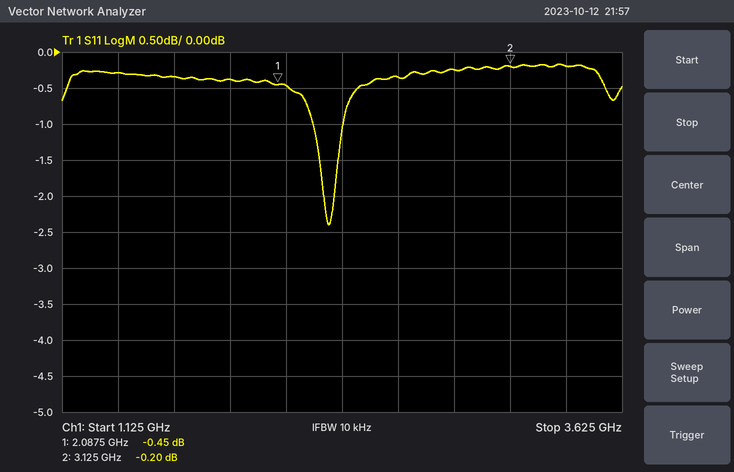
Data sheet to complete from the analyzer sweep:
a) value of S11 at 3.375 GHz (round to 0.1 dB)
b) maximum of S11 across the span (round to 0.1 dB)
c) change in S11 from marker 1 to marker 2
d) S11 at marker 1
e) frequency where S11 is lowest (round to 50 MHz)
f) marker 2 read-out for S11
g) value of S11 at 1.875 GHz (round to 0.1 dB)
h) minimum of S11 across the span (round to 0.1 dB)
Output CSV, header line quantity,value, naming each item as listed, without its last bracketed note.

quantity,value
value of S11 at 3.375 GHz,-0.2 dB
maximum of S11 across the span,-0.2 dB
change in S11 from marker 1 to marker 2,0.25 dB
S11 at marker 1,-0.45 dB
frequency where S11 is lowest,2.30 GHz
marker 2 read-out for S11,-0.20 dB
value of S11 at 1.875 GHz,-0.4 dB
minimum of S11 across the span,-2.4 dB
